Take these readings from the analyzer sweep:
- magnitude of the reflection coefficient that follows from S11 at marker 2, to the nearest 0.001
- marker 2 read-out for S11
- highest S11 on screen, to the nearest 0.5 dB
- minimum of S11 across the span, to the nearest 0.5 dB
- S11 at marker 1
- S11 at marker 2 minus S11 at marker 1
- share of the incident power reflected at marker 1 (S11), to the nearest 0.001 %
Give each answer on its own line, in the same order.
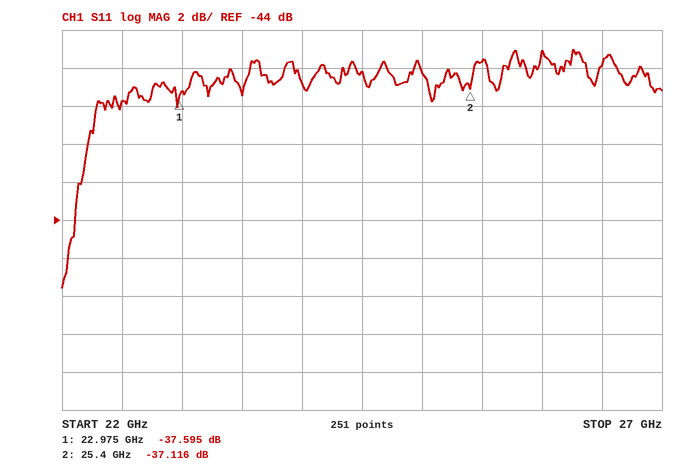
0.014
-37.116 dB
-35.0 dB
-47.5 dB
-37.595 dB
0.479 dB
0.017 %
